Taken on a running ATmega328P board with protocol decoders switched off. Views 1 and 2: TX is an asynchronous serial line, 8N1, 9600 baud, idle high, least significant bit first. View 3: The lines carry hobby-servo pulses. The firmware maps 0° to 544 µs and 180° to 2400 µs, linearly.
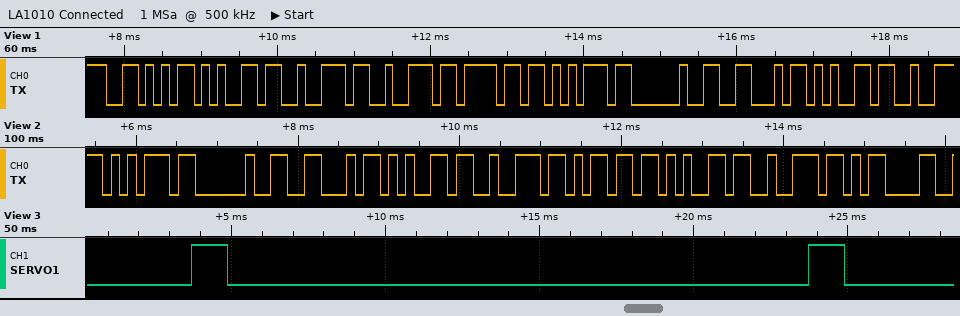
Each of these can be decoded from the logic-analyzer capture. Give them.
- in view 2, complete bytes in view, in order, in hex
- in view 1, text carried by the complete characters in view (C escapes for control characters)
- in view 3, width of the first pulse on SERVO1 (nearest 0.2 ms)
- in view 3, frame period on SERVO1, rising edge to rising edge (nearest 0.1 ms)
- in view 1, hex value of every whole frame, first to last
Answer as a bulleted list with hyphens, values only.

- 75 20 46 65 72 6D 65 72 0D
- "Verrou Fe"
- 1.2 ms
- 20.0 ms
- 0x56 0x65 0x72 0x72 0x6F 0x75 0x20 0x46 0x65
